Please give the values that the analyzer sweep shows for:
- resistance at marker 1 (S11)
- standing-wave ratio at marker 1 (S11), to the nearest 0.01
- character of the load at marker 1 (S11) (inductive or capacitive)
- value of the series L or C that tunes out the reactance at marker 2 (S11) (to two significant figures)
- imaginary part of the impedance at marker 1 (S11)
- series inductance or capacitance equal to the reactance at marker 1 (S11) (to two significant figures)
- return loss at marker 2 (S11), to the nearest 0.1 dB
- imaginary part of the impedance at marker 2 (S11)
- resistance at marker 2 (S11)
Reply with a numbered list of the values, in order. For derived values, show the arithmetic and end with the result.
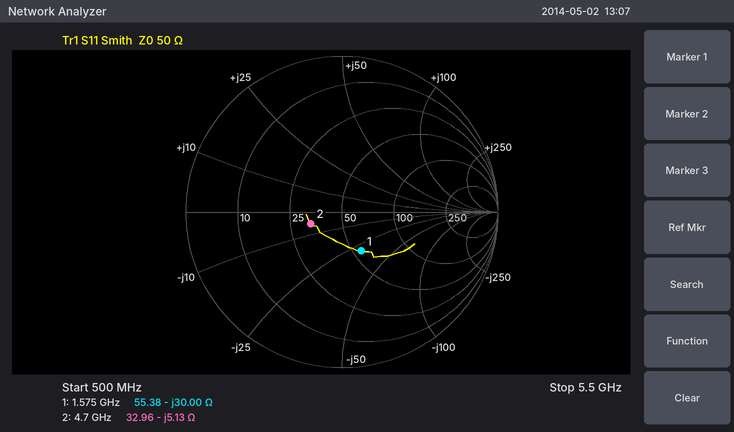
1. 55.38 Ω
2. 1.77
3. capacitive
4. L = 5.13 Ω/(2π × 4.7 GHz) ≈ 174 pH, so 170 pH to two significant figures
5. -30.00 Ω
6. C = 1/(2π × 1.575 GHz × 30 Ω) ≈ 3.4 pF
7. 13.4 dB
8. -5.13 Ω
9. 32.96 Ω
